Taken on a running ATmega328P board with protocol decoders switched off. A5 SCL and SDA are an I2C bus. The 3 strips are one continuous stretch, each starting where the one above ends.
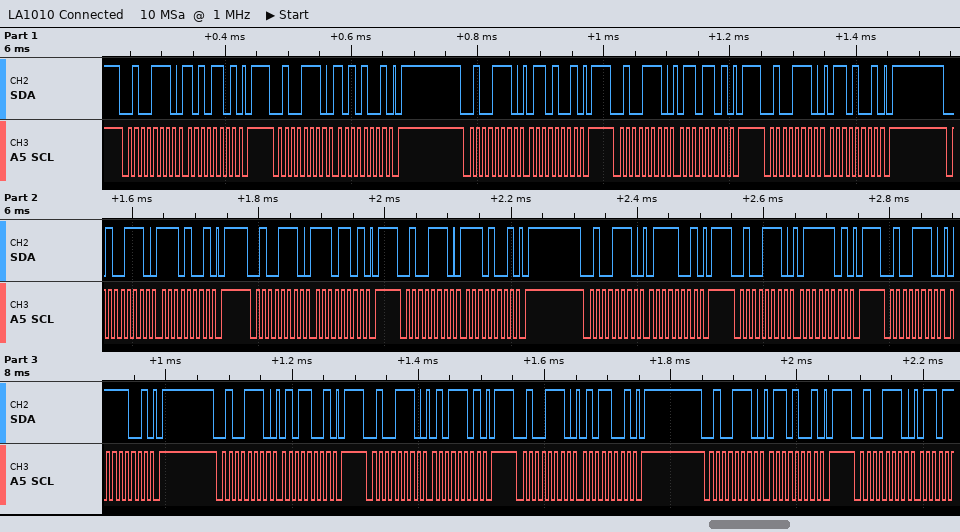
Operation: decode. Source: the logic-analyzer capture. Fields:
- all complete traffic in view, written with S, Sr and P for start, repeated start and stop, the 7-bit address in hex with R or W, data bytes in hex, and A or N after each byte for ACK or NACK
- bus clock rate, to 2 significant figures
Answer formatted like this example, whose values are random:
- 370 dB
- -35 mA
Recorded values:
- S 27W A AD A P S 27W A A9 A P S 27W A 69 A P S 27W A 6D A P S 27W A 69 A P S 27W A E9 A P S 27W A ED A P S 27W A E9 A P S 27W A 79 A P S 27W A 7D A P S 27W A 79 A P S 27W A 59 A P S 27W A 5D A P S 27W A 59 A P S 27W A 69 A P S 27W A
- 100 kHz
